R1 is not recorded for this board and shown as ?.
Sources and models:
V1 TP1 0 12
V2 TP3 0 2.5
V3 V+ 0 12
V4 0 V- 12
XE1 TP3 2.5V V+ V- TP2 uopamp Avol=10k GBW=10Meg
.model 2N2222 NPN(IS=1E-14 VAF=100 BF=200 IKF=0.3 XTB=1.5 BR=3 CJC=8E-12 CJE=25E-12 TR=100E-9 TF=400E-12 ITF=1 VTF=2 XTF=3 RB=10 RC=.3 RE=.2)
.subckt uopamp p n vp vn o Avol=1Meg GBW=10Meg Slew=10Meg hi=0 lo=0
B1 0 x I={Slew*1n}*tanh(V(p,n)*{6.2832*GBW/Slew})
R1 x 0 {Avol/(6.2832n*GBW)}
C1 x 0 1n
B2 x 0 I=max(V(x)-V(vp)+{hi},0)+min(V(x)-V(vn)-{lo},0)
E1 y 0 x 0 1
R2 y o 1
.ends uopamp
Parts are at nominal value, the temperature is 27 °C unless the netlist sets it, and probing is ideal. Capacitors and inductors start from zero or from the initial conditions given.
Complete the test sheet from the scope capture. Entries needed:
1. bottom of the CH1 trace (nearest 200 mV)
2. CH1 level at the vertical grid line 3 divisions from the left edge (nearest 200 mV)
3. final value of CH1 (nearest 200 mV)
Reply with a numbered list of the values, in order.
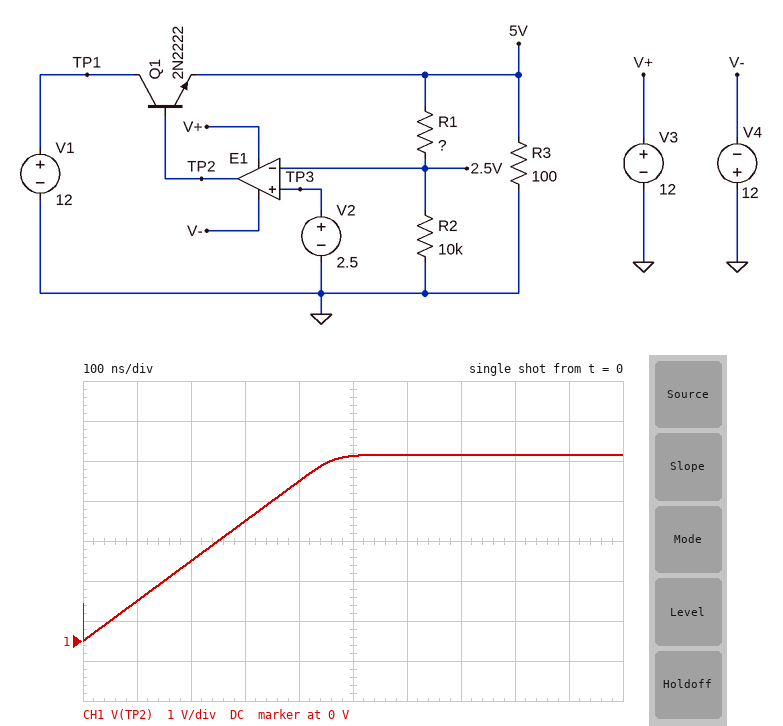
1. 0 V
2. 3.0 V
3. 4.6 V
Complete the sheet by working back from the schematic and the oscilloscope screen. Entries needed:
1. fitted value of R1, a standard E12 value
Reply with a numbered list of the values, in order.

1. 5.6 kΩ
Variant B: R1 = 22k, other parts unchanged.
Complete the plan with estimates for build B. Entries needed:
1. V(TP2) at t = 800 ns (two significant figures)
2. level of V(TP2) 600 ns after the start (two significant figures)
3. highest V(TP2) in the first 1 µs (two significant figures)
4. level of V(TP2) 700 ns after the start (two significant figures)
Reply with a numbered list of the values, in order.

1. 8.0 V
2. 6.0 V
3. 8.8 V
4. 7.0 V
